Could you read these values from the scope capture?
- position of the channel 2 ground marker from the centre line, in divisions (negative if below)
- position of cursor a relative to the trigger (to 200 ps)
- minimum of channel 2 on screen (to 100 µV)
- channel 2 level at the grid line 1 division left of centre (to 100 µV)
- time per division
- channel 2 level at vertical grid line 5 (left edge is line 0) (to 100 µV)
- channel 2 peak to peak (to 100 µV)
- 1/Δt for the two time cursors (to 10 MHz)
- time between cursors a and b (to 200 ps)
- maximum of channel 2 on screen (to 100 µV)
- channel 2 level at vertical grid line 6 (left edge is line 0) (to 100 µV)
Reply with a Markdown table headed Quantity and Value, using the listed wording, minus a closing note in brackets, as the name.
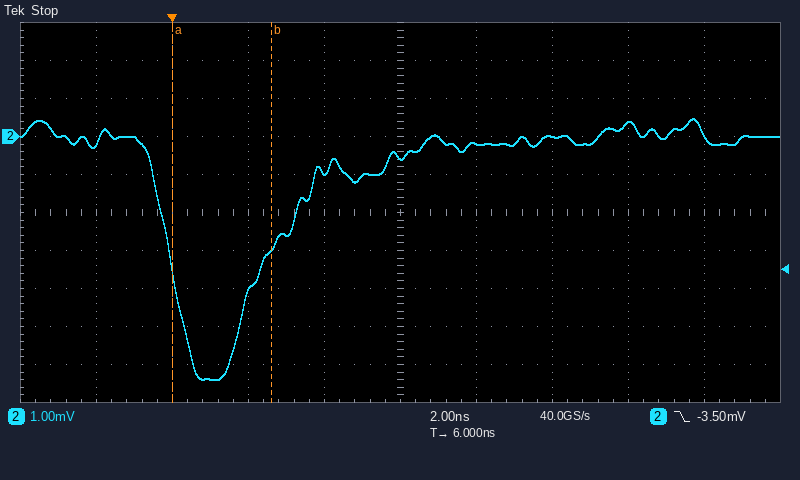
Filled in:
| Quantity | Value |
|---|---|
| position of the channel 2 ground marker from the centre line, in divisions | +2.0 div |
| position of cursor a relative to the trigger | 0.0 ns |
| minimum of channel 2 on screen | -6.4 mV |
| channel 2 level at the grid line 1 division left of centre | -900 µV |
| time per division | 2 ns |
| channel 2 level at vertical grid line 5 (left edge is line 0) | -500 µV |
| channel 2 peak to peak | 6.9 mV |
| 1/Δt for the two time cursors | 380 MHz |
| time between cursors a and b | 2.6 ns |
| maximum of channel 2 on screen | 500 µV |
| channel 2 level at vertical grid line 6 (left edge is line 0) | -200 µV |
